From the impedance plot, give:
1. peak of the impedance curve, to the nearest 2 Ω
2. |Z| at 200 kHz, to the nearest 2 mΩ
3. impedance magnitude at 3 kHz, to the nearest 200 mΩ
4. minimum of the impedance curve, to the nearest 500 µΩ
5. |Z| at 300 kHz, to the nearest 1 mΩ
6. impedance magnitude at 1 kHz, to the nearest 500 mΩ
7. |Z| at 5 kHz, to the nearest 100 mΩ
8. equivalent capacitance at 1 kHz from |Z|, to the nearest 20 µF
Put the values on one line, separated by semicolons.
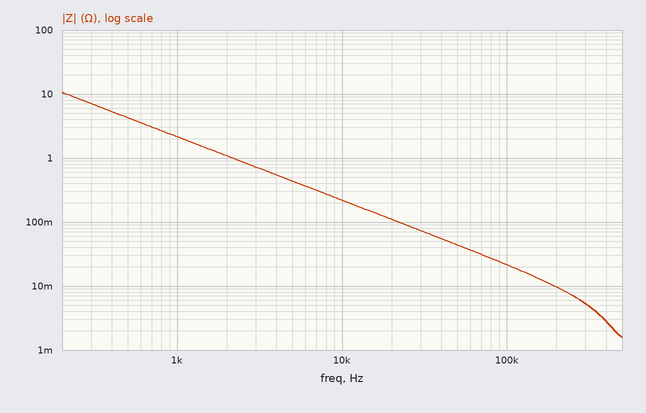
10 Ω; 10 mΩ; 800 mΩ; 1.5 mΩ; 5 mΩ; 2.0 Ω; 400 mΩ; 80 µF
